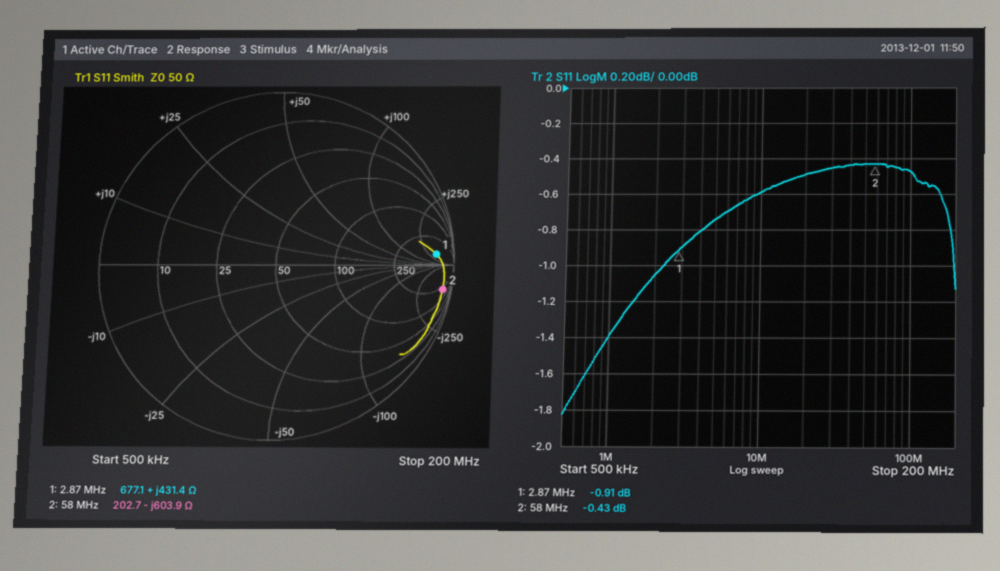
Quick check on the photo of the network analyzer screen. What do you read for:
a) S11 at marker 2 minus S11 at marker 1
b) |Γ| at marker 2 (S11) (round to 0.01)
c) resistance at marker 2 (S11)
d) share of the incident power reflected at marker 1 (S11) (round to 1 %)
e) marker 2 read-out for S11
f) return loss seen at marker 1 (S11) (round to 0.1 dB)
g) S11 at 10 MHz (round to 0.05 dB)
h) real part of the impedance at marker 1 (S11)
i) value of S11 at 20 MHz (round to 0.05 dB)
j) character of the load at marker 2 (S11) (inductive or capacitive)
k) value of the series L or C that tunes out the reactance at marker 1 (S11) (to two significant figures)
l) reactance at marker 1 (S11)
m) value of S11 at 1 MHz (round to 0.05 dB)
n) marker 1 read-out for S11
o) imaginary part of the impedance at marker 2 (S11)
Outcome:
0.48 dB
0.95
202.7 Ω
81 %
-0.43 dB
0.9 dB
-0.60 dB
677.1 Ω
-0.50 dB
capacitive
130 pF
+431.4 Ω
-1.40 dB
-0.91 dB
-603.9 Ω
